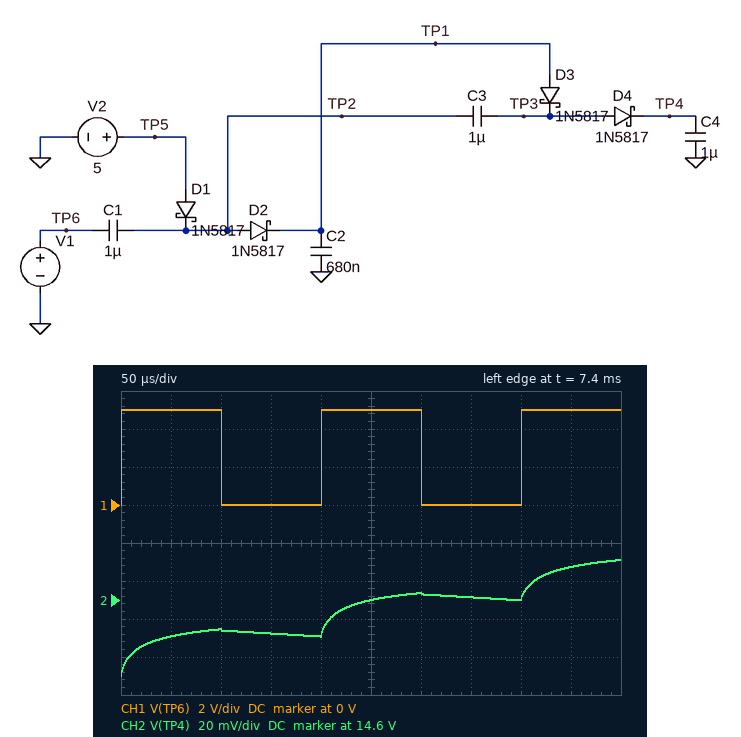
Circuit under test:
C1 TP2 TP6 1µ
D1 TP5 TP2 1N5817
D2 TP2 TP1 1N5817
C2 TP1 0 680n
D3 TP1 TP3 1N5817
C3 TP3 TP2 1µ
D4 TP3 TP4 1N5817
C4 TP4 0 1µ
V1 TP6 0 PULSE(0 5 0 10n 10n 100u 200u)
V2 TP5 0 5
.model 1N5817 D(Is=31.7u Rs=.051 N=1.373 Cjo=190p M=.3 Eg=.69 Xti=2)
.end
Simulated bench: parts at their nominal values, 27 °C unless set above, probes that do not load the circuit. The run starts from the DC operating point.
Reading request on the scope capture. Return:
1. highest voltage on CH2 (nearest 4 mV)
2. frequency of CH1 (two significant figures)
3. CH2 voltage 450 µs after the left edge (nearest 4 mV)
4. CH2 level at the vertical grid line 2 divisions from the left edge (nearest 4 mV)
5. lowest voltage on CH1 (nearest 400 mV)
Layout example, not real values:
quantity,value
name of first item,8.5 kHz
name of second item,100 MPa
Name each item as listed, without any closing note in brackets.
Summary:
quantity,value
highest voltage on CH2,14.620 V
frequency of CH1,5.0 kHz
CH2 voltage 450 µs after the left edge,14.616 V
CH2 level at the vertical grid line 2 divisions from the left edge,14.584 V
lowest voltage on CH1,0 V
